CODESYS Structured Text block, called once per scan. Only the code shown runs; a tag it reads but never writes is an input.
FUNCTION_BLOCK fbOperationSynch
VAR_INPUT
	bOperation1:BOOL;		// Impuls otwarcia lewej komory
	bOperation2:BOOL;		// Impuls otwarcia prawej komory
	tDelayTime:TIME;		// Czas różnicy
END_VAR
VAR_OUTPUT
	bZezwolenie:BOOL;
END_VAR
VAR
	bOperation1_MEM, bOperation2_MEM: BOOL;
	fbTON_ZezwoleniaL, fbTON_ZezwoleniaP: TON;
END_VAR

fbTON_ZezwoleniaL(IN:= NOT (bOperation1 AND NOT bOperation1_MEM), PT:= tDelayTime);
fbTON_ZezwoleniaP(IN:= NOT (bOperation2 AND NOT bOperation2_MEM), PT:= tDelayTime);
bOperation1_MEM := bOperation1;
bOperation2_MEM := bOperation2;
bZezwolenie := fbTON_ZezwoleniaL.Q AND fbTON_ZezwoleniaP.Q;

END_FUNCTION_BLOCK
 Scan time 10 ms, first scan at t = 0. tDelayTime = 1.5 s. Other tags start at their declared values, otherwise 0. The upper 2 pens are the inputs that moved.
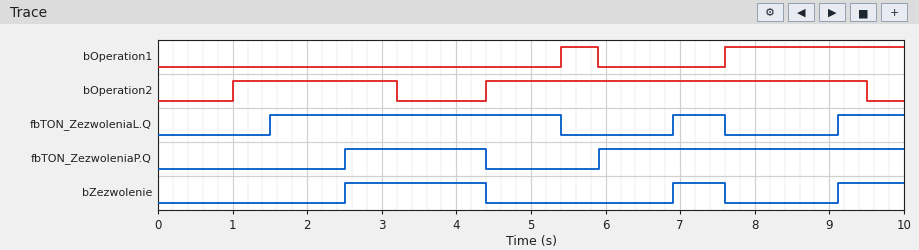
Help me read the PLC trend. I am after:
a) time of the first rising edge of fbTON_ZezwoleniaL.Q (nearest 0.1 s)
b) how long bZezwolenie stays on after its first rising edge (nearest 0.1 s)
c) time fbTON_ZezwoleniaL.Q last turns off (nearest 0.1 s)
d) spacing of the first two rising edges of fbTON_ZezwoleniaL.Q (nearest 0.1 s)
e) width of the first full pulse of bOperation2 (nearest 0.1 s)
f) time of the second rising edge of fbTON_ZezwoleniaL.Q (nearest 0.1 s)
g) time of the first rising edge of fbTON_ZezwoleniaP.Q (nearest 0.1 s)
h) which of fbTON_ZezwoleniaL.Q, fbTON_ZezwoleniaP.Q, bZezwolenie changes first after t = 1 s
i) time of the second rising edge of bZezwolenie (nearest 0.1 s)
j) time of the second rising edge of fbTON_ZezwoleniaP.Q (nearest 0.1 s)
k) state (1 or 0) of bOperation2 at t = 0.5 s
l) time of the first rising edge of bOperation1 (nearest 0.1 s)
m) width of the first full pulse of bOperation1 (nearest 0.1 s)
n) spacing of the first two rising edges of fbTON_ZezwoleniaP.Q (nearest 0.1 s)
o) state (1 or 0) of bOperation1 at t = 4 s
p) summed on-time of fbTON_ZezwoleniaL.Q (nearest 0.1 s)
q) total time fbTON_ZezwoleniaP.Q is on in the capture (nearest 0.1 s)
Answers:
1.5 s
1.9 s
7.6 s
5.4 s
2.2 s
6.9 s
2.5 s
fbTON_ZezwoleniaL.Q
6.9 s
5.9 s
0
5.4 s
0.5 s
3.4 s
0
5.5 s
6.0 s
